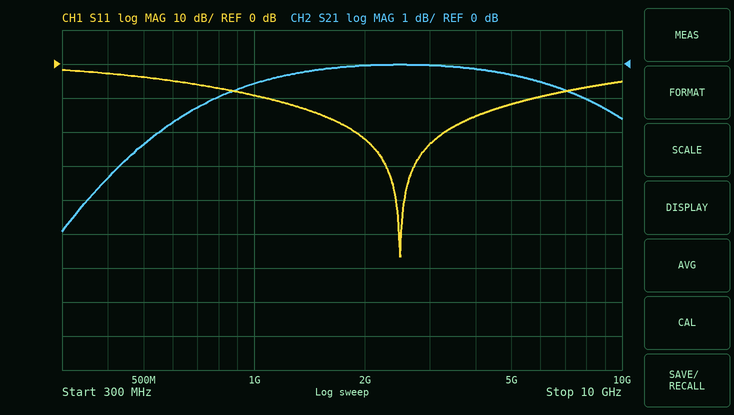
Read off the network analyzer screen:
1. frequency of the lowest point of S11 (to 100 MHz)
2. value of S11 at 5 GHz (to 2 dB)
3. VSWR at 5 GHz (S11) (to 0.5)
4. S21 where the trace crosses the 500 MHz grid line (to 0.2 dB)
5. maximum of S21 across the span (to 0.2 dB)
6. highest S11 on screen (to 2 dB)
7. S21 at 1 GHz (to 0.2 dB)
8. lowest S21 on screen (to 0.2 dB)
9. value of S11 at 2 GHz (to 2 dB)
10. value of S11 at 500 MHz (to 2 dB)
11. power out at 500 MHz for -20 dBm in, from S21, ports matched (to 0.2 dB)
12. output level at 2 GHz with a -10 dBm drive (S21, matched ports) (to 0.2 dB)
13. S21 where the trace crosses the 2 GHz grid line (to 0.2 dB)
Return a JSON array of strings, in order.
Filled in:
["2.5 GHz", "-12 dB", "1.5", "-2.4 dB", "0.0 dB", "-2 dB", "-0.6 dB", "-5.0 dB", "-22 dB", "-4 dB", "-22.4 dBm", "-10.0 dBm", "0.0 dB"]
